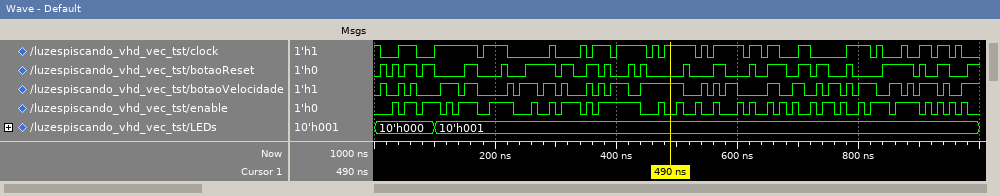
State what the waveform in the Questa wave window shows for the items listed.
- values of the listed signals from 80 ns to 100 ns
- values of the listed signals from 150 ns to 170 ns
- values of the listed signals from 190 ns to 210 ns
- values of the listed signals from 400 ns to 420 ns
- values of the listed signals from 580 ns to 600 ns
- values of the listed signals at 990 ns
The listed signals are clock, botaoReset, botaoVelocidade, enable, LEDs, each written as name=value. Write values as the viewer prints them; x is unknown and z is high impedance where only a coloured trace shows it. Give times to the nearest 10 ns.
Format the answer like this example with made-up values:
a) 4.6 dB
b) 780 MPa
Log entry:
a) clock=0, botaoReset=1, botaoVelocidade=0, enable=1, LEDs=10'h000
b) clock=1, botaoReset=1, botaoVelocidade=1, enable=1, LEDs=10'h001
c) clock=1, botaoReset=0, botaoVelocidade=0, enable=1, LEDs=10'h001
d) clock=1, botaoReset=0, botaoVelocidade=1, enable=1, LEDs=10'h001
e) clock=1, botaoReset=0, botaoVelocidade=1, enable=0, LEDs=10'h001
f) clock=0, botaoReset=1, botaoVelocidade=1, enable=0, LEDs=10'h001
